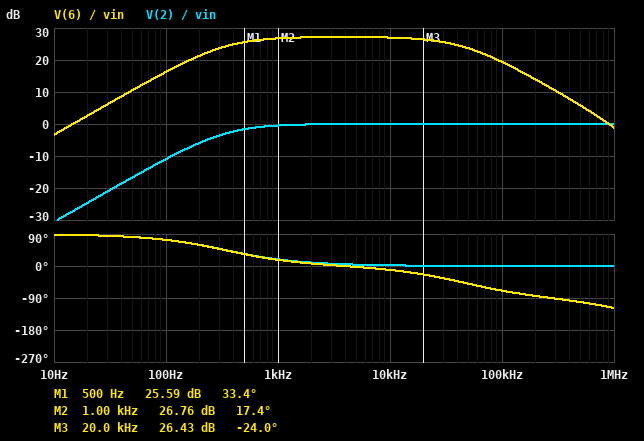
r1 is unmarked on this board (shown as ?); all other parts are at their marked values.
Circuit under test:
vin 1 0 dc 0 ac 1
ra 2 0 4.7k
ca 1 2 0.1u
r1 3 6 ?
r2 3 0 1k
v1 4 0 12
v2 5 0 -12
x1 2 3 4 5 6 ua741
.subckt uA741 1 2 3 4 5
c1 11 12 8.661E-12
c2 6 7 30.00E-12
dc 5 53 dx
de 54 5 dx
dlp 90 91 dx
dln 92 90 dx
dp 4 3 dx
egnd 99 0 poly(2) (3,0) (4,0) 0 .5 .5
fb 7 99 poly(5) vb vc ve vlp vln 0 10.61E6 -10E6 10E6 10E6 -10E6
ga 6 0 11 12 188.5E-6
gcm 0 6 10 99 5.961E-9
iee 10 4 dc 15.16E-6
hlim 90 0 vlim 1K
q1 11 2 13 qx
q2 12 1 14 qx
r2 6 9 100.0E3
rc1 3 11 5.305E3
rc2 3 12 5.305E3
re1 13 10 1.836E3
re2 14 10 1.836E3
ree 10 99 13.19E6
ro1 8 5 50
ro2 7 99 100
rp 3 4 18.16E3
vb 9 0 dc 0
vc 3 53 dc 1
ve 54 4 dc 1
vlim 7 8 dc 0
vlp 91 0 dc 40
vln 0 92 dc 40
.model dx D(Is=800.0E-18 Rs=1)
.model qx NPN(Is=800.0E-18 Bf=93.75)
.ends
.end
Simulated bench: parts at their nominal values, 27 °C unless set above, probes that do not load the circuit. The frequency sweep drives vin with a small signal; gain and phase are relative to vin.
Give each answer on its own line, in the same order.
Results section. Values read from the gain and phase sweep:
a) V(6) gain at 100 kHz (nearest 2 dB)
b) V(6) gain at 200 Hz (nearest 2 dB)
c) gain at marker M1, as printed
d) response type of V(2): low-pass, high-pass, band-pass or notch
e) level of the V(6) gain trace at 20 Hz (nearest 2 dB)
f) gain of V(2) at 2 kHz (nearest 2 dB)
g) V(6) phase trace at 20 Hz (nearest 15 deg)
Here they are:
20 dB
22 dB
25.59 dB
high-pass
2 dB
0 dB
90 deg
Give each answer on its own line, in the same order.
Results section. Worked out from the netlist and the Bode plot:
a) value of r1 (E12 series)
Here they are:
22 kΩ
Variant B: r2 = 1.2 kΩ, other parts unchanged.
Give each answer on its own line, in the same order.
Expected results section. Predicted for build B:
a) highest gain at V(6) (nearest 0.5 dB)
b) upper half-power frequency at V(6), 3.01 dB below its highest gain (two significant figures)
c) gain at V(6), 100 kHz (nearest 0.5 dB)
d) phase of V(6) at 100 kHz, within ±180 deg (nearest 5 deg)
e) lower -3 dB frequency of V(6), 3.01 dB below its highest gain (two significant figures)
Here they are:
25.5 dB
54 kHz
19.0 dB
-65 deg
330 Hz
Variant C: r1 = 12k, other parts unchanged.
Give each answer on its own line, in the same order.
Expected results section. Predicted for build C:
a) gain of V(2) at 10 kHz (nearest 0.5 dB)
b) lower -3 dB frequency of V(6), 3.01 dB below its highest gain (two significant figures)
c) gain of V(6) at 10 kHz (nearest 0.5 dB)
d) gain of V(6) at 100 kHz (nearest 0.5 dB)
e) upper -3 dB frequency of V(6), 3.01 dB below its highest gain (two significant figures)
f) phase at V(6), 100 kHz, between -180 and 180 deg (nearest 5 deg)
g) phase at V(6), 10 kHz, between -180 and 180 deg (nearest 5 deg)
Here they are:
0 dB
340 Hz
22.0 dB
18.0 dB
81 kHz
-55 deg
-5 deg
